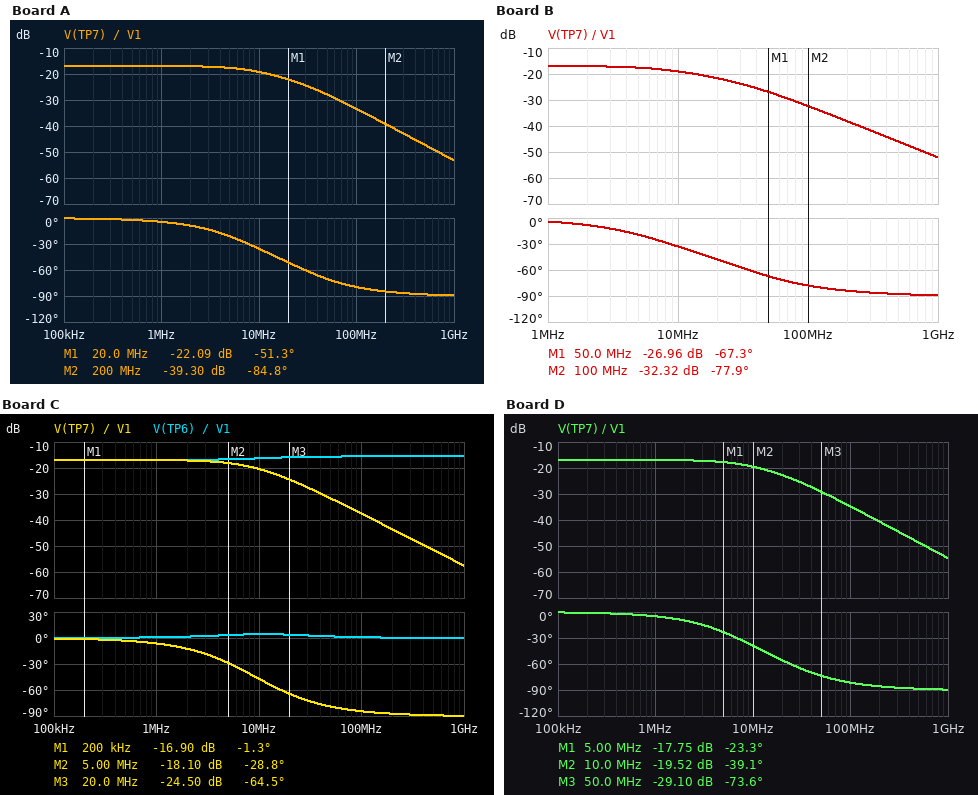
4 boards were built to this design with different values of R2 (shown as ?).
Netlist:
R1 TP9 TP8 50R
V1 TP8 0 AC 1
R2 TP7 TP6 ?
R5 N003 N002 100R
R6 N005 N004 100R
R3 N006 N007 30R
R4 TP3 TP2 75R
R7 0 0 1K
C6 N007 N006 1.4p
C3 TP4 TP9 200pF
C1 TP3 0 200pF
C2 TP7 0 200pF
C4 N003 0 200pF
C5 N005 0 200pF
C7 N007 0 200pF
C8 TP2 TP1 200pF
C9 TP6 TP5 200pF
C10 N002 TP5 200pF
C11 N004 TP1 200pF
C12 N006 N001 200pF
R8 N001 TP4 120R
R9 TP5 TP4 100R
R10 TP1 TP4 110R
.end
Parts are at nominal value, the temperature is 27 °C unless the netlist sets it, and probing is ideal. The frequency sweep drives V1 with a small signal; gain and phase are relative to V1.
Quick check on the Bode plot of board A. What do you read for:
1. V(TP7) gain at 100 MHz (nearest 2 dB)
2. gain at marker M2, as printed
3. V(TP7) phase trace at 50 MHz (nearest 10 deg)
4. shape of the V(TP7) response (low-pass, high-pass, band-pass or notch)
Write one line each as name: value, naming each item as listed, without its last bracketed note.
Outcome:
V(TP7) gain at 100 MHz: -34 dB
gain at marker M2, as printed: -39.30 dB
V(TP7) phase trace at 50 MHz: -70 deg
shape of the V(TP7) response: low-pass
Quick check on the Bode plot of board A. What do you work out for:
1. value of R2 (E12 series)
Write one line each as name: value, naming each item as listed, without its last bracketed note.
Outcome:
value of R2: 39 Ω
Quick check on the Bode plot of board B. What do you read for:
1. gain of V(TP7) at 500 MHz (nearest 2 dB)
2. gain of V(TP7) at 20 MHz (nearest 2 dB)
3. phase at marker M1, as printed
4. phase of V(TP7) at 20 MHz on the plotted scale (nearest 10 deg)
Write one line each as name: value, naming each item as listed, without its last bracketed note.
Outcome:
gain of V(TP7) at 500 MHz: -46 dB
gain of V(TP7) at 20 MHz: -22 dB
phase at marker M1, as printed: -67.3 deg
phase of V(TP7) at 20 MHz on the plotted scale: -50 deg
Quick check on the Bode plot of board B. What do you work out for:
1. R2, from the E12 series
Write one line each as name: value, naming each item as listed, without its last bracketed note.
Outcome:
R2, from the E12 series: 27 Ω
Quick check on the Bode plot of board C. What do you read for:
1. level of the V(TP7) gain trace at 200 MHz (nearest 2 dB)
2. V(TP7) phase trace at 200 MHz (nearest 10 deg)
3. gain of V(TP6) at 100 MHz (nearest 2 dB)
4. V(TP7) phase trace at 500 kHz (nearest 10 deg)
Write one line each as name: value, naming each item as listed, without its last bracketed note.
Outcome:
level of the V(TP7) gain trace at 200 MHz: -44 dB
V(TP7) phase trace at 200 MHz: -90 deg
gain of V(TP6) at 100 MHz: -16 dB
V(TP7) phase trace at 500 kHz: 0 deg
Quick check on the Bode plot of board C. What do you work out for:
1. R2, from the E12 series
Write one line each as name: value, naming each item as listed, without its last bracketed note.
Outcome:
R2, from the E12 series: 100 Ω
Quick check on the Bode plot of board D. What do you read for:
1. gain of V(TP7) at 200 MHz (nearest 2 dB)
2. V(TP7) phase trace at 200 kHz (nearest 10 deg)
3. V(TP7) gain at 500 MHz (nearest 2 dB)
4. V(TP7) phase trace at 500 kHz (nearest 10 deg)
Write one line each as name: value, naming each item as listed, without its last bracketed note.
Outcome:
gain of V(TP7) at 200 MHz: -40 dB
V(TP7) phase trace at 200 kHz: 0 deg
V(TP7) gain at 500 MHz: -48 dB
V(TP7) phase trace at 500 kHz: 0 deg
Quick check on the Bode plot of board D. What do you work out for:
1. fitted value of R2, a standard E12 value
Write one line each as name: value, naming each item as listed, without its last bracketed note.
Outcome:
fitted value of R2, a standard E12 value: 56 Ω
